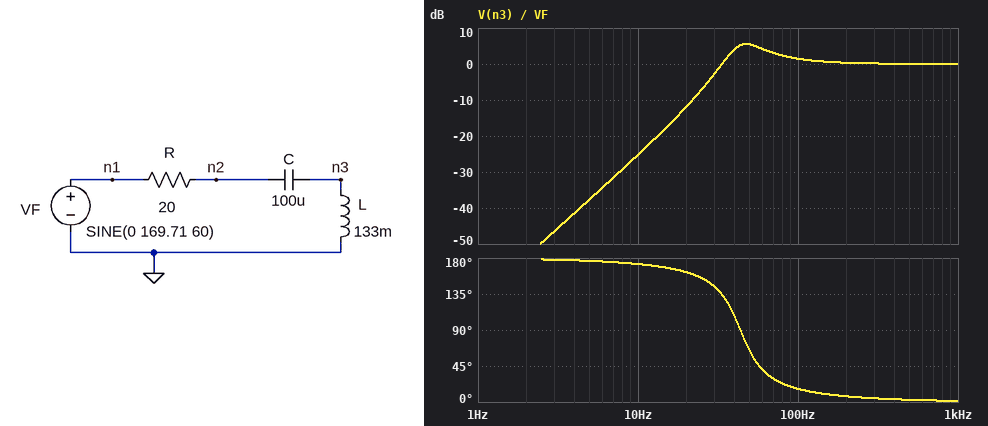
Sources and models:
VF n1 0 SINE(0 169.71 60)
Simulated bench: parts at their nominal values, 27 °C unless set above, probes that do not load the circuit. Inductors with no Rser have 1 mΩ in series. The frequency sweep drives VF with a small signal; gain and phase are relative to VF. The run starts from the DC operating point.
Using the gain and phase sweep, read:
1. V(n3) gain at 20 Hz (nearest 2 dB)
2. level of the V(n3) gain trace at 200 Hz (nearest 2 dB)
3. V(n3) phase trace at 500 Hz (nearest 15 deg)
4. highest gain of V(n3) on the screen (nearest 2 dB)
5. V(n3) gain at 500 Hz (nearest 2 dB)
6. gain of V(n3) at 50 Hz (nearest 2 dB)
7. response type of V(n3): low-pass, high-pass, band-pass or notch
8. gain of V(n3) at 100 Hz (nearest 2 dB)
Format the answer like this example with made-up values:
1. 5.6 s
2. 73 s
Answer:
1. -12 dB
2. 0 dB
3. 0 deg
4. 6 dB
5. 0 dB
6. 6 dB
7. high-pass
8. 2 dB
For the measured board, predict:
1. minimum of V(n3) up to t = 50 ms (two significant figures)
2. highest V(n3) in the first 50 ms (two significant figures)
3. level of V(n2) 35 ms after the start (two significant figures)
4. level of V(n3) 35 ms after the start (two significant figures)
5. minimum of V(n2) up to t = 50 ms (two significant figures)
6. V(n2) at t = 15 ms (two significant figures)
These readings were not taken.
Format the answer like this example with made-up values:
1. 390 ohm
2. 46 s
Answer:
1. -300 V
2. 290 V
3. 130 V
4. 280 V
5. -130 V
6. 10 V
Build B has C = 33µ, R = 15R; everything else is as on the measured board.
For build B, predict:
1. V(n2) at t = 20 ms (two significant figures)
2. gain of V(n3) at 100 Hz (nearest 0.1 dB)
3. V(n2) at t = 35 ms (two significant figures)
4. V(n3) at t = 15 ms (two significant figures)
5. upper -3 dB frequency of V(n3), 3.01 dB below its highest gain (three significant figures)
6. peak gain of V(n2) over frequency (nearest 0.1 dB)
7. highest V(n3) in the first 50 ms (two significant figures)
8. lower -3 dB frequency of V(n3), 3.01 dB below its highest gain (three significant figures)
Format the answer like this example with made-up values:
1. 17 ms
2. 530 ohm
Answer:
1. 86 V
2. 6.8 dB
3. 16 V
4. 290 V
5. 88.5 Hz
6. 0 dB
7. 310 V
8. 69.2 Hz
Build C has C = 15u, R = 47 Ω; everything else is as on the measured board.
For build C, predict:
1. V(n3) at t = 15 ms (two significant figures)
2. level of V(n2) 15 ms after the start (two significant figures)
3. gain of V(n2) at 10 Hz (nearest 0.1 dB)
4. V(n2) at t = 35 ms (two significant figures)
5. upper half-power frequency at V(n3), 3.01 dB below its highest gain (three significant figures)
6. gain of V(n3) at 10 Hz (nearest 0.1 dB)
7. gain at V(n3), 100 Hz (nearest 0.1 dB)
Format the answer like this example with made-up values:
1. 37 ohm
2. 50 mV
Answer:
1. 47 V
2. -140 V
3. 0 dB
4. 43 V
5. 180 Hz
6. -42.0 dB
7. 4.1 dB
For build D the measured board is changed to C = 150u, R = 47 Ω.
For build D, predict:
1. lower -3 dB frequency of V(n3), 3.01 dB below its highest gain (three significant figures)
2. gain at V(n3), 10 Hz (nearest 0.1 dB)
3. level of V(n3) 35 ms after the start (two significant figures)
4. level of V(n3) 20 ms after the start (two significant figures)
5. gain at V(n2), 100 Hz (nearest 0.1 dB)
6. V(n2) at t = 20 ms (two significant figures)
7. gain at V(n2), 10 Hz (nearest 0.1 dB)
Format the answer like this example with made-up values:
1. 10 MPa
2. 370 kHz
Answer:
1. 40.2 Hz
2. -22.3 dB
3. 150 V
4. 120 V
5. -1.5 dB
6. 81 V
7. -0.9 dB
